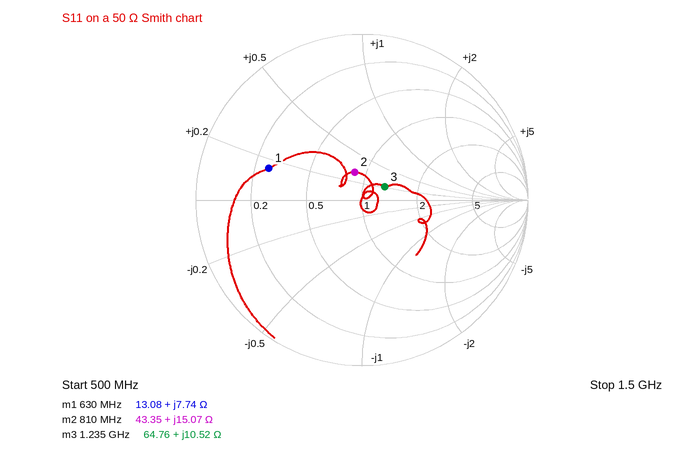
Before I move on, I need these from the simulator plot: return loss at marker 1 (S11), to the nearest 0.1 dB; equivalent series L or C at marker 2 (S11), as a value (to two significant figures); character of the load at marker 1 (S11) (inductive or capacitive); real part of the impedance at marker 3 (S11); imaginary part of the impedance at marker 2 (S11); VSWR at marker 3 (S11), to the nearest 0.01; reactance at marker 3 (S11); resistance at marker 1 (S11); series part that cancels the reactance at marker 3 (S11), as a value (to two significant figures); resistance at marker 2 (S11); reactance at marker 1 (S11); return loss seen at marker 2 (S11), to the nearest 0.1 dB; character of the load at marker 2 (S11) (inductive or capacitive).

4.5 dB
3.0 nH
inductive
64.76 Ω
+15.07 Ω
1.37
+10.52 Ω
13.08 Ω
12 pF
43.35 Ω
+7.74 Ω
15.2 dB
inductive
